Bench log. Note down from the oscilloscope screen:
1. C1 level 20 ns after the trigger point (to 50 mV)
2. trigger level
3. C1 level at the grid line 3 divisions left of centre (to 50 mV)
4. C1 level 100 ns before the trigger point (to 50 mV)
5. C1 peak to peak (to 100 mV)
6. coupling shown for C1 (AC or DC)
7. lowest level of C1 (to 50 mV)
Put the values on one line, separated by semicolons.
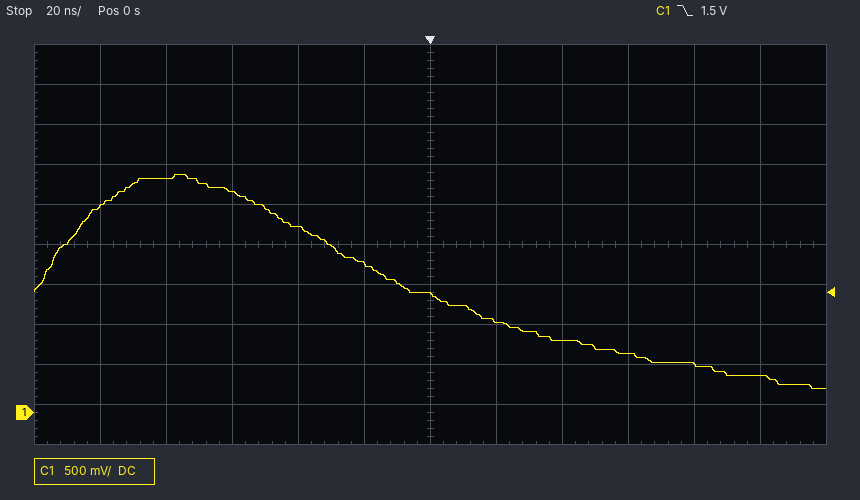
1.15 V; 1.5 V; 2.75 V; 2.55 V; 2.70 V; DC; 300 mV
